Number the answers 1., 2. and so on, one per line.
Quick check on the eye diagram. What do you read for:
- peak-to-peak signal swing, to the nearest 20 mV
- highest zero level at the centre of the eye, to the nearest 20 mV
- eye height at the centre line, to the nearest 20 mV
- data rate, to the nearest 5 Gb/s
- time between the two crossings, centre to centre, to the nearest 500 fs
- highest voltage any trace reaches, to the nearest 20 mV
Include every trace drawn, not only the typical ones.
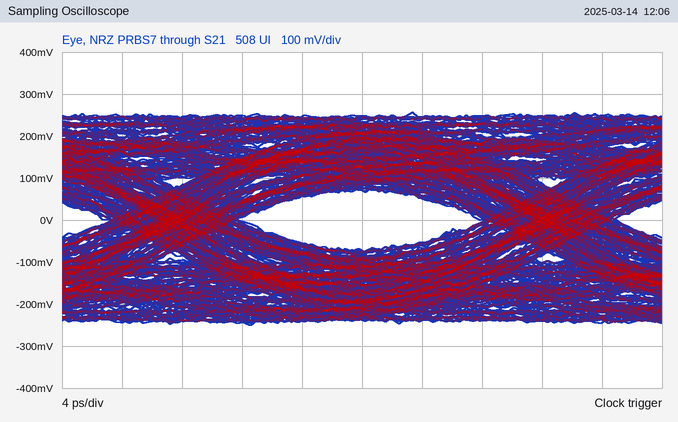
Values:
1. 500 mV
2. -80 mV
3. 140 mV
4. 40 Gb/s
5. 25.0 ps
6. 260 mV
